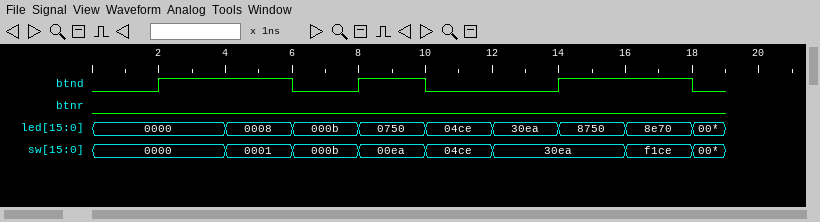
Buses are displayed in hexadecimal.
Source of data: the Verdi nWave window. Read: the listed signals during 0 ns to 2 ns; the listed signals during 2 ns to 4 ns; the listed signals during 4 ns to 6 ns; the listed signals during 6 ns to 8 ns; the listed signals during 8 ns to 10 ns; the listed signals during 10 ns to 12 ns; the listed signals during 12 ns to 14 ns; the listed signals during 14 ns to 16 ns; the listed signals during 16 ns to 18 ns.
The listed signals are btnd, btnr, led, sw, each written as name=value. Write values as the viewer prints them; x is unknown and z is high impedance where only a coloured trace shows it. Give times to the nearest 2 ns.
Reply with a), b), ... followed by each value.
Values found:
a) btnd=0, btnr=0, led=0000, sw=0000
b) btnd=1, btnr=0, led=0000, sw=0000
c) btnd=1, btnr=0, led=0008, sw=0001
d) btnd=0, btnr=0, led=000b, sw=000b
e) btnd=1, btnr=0, led=0750, sw=00ea
f) btnd=0, btnr=0, led=04ce, sw=04ce
g) btnd=0, btnr=0, led=30ea, sw=30ea
h) btnd=1, btnr=0, led=8750, sw=30ea
i) btnd=1, btnr=0, led=8e70, sw=f1ce
